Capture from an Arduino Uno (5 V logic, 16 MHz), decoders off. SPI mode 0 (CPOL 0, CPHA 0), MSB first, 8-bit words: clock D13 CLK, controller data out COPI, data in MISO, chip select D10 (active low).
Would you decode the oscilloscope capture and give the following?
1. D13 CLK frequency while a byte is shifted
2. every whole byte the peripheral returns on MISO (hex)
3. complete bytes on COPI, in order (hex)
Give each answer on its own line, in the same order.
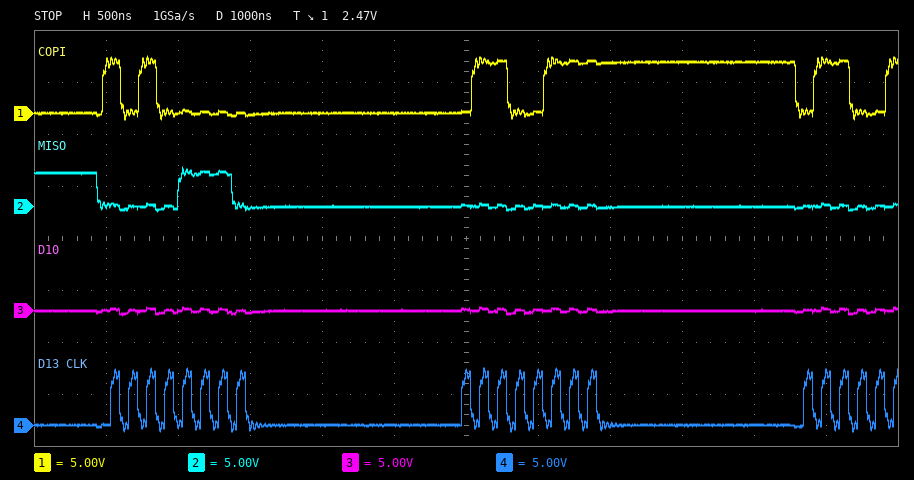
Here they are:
8 MHz
0E 00
A0 67
